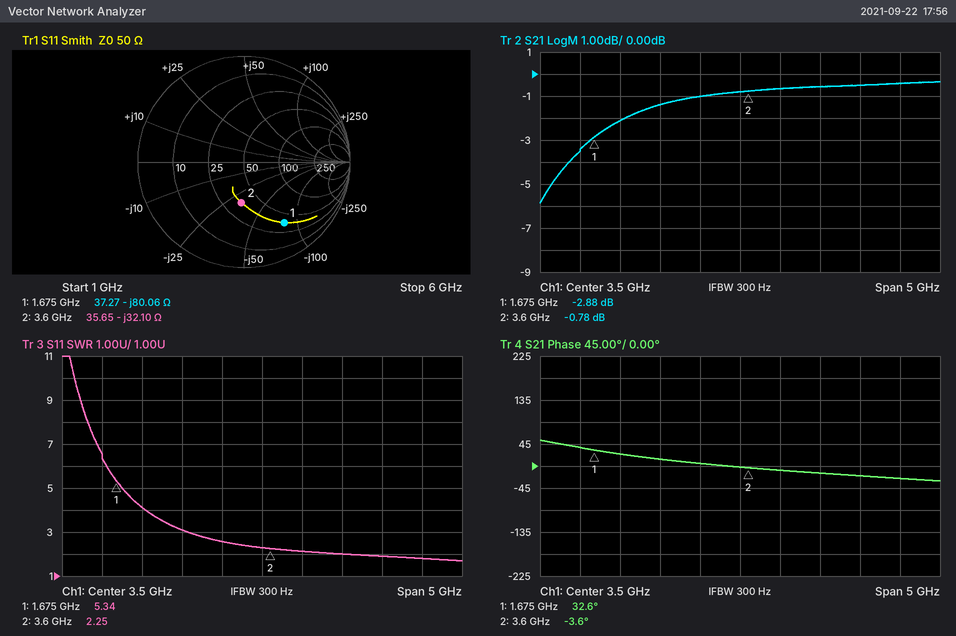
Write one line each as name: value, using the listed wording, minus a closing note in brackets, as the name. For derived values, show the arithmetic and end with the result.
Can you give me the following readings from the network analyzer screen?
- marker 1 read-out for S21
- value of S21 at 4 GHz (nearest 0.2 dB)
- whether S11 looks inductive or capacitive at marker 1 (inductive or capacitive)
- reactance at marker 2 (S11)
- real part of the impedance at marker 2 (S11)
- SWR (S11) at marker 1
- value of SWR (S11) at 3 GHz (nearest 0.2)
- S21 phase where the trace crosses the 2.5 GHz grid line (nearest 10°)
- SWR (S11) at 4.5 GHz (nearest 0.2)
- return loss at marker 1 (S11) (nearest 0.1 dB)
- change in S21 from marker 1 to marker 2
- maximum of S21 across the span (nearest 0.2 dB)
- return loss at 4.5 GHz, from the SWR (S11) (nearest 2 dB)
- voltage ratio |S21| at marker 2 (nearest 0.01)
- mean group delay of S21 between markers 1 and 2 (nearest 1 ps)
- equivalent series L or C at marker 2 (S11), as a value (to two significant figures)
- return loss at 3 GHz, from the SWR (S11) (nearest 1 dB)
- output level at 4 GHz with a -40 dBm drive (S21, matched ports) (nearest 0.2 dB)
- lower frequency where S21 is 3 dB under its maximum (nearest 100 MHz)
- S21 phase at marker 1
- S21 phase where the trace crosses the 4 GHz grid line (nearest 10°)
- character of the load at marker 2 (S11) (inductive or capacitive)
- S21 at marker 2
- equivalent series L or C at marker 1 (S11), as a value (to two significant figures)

marker 1 read-out for S21: -2.88 dB
value of S21 at 4 GHz: -0.6 dB
whether S11 looks inductive or capacitive at marker 1: capacitive
reactance at marker 2: -32.10 Ω
real part of the impedance at marker 2: 35.65 Ω
SWR (S11) at marker 1: 5.34
value of SWR (S11) at 3 GHz: 2.6
S21 phase where the trace crosses the 2.5 GHz grid line: 10°
SWR (S11) at 4.5 GHz: 2.0
return loss at marker 1 (S11): 3.3 dB
change in S21 from marker 1 to marker 2: -0.78 − (-2.88) = 2.10 dB
maximum of S21 across the span: -0.4 dB
return loss at 4.5 GHz, from the SWR (S11): −20 log10((2 − 1)/(2 + 1)) ≈ 10 dB
voltage ratio |S21| at marker 2: 10^(-0.78/20) ≈ 0.91
mean group delay of S21 between markers 1 and 2: −(-3.6° − (32.6°))/(360° × 1.925 GHz) ≈ 52 ps
equivalent series L or C at marker 2 (S11), as a value: C = 1/(2π × 3.6 GHz × 32.1 Ω) ≈ 1.4 pF
return loss at 3 GHz, from the SWR (S11): −20 log10((2.6 − 1)/(2.6 + 1)) ≈ 7 dB
output level at 4 GHz with a -40 dBm drive (S21, matched ports): -40 dBm + (-0.6 dB) = -40.6 dBm
lower frequency where S21 is 3 dB under its maximum: 1.5 GHz
S21 phase at marker 1: 32.6°
S21 phase where the trace crosses the 4 GHz grid line: -10°
character of the load at marker 2 (S11): capacitive
S21 at marker 2: -0.78 dB
equivalent series L or C at marker 1 (S11), as a value: C = 1/(2π × 1.675 GHz × 80.06 Ω) ≈ 1.2 pF
